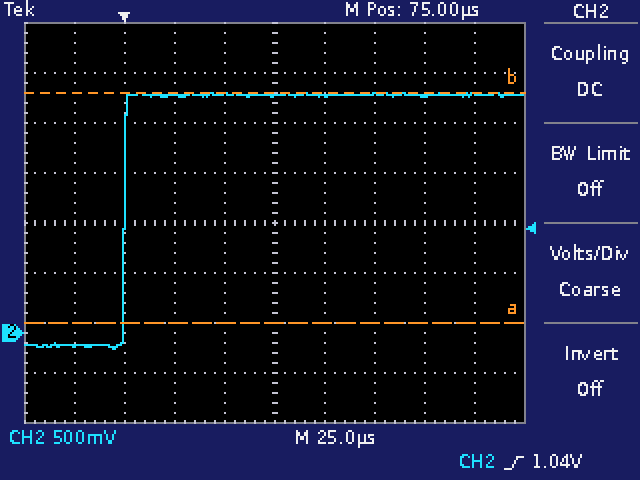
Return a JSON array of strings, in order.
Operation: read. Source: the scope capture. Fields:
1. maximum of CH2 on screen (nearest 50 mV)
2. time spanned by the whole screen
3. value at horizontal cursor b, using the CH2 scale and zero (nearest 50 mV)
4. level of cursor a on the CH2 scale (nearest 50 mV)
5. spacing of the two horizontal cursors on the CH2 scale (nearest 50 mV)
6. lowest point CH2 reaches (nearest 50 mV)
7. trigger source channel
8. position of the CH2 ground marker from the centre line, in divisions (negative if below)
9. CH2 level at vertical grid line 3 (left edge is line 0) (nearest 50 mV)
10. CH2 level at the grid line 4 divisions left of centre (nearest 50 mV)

["2.40 V", "250 µs", "2.40 V", "100 mV", "2.30 V", "-150 mV", "CH2", "-2.2 div", "2.40 V", "-150 mV"]
